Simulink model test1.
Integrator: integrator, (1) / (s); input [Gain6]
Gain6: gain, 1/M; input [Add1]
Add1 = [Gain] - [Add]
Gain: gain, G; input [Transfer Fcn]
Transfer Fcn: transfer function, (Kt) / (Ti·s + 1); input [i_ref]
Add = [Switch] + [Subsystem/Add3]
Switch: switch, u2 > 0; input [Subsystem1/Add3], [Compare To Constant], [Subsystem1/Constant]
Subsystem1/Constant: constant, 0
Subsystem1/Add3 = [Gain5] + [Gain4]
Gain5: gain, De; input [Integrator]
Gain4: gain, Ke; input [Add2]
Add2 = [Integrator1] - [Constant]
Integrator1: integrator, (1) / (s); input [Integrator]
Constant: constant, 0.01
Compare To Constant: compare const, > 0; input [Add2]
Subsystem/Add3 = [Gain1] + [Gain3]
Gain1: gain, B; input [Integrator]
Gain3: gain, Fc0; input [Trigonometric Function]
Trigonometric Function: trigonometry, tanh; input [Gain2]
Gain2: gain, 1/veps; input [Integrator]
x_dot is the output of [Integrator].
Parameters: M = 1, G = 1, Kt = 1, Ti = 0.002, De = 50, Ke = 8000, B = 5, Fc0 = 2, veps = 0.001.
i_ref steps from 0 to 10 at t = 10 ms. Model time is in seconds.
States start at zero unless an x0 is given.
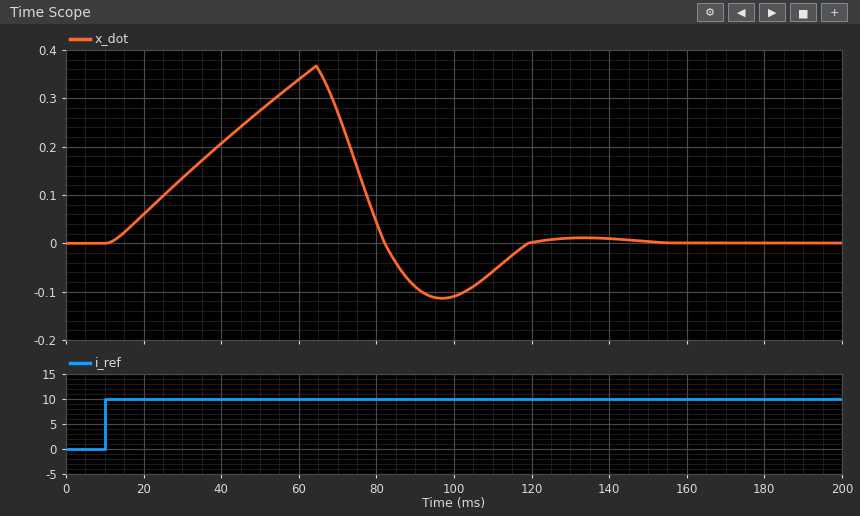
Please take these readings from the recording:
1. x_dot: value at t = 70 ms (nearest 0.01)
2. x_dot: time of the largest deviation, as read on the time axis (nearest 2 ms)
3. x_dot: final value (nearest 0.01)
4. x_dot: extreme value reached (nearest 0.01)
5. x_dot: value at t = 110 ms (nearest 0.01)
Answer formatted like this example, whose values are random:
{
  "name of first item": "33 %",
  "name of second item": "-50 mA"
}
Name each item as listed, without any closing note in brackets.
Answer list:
{
  "x_dot: value at t = 70 ms": "0.27",
  "x_dot: time of the largest deviation, as read on the time axis": "64 ms",
  "x_dot: final value": "0.00",
  "x_dot: extreme value reached": "0.37",
  "x_dot: value at t = 110 ms": "-0.06"
}
